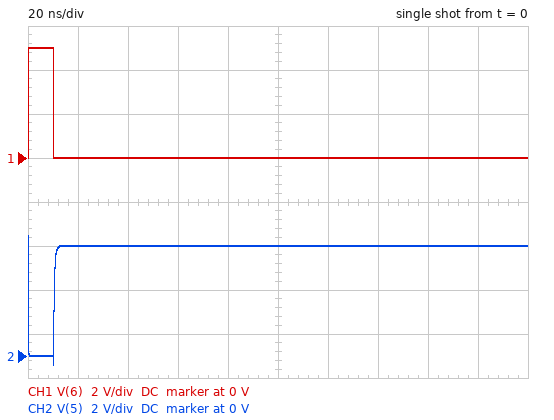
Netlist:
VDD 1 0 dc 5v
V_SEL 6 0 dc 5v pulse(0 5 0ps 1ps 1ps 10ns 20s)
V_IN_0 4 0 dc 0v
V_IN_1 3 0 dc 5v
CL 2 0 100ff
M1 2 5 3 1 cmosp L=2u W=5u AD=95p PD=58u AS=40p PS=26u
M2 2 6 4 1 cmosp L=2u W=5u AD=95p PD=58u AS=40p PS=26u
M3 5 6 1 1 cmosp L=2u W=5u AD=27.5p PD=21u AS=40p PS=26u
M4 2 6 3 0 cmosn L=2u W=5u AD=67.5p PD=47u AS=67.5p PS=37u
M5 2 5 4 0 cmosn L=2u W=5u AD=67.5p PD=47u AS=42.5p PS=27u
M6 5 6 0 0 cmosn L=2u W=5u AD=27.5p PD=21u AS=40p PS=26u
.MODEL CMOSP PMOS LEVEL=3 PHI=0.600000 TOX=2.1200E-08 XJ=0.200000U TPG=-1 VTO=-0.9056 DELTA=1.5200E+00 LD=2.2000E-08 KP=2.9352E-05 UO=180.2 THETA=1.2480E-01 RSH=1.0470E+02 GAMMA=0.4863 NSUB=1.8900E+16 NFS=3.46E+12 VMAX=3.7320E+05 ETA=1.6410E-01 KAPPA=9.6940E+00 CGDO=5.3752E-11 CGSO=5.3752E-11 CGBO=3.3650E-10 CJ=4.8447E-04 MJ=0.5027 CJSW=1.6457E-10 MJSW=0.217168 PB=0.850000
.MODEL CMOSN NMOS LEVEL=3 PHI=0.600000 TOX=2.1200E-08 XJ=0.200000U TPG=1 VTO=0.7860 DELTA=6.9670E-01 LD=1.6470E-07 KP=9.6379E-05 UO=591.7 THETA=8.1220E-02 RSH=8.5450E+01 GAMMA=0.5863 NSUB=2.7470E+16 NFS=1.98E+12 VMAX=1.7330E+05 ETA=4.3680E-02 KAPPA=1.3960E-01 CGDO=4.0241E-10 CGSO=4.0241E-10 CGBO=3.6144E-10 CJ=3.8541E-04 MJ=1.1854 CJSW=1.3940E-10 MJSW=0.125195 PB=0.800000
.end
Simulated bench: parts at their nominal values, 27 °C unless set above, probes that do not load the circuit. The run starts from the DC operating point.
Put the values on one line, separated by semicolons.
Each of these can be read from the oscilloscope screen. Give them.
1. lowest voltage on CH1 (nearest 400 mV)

0 V
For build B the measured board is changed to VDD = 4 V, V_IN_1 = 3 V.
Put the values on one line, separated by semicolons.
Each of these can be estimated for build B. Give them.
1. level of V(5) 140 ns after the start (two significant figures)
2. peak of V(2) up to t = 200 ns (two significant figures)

4.0 V; 3.0 V
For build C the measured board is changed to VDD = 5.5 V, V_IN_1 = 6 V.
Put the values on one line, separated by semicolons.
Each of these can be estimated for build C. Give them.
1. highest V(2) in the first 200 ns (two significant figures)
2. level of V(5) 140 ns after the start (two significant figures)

6.0 V; 5.5 V
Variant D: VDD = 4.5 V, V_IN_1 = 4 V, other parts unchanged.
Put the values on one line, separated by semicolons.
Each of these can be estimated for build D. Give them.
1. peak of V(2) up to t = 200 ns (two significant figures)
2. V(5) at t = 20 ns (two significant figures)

4.0 V; 4.5 V
